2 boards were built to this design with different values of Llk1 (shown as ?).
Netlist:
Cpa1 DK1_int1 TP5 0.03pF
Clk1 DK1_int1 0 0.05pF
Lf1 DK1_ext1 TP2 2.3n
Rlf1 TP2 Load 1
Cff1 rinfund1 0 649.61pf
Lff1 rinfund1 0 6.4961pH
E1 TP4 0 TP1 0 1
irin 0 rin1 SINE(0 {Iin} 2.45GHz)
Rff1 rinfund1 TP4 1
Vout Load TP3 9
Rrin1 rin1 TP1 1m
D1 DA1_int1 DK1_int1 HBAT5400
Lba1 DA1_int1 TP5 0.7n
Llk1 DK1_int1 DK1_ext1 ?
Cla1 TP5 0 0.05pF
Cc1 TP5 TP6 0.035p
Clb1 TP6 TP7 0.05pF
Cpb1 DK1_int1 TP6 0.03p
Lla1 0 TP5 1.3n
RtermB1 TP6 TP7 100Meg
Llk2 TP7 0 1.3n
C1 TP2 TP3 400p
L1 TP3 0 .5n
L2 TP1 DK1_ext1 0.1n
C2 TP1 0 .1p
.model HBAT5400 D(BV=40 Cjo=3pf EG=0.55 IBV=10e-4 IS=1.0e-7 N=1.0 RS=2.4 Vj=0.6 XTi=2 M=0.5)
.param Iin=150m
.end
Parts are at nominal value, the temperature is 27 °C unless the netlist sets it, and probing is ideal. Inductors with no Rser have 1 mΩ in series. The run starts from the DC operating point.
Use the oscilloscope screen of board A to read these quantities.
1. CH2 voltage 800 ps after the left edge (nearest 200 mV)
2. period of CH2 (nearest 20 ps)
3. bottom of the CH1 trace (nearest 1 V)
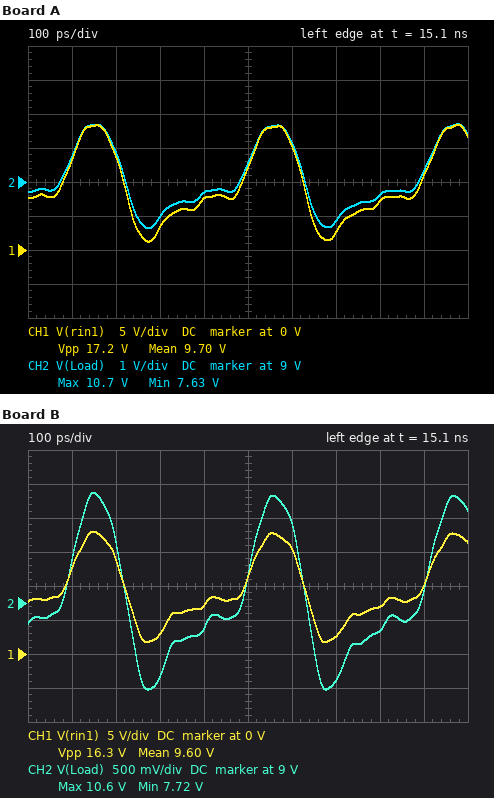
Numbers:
8.6 V
400 ps
1 V
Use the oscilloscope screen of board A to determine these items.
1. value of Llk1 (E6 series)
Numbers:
330 pH
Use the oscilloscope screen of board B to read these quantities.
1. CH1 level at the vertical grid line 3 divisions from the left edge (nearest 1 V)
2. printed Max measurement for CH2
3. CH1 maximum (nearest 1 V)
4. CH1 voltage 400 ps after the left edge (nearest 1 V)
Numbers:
3 V
10.6 V
18 V
7 V
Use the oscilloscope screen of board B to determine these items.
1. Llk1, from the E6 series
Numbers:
470 pH
